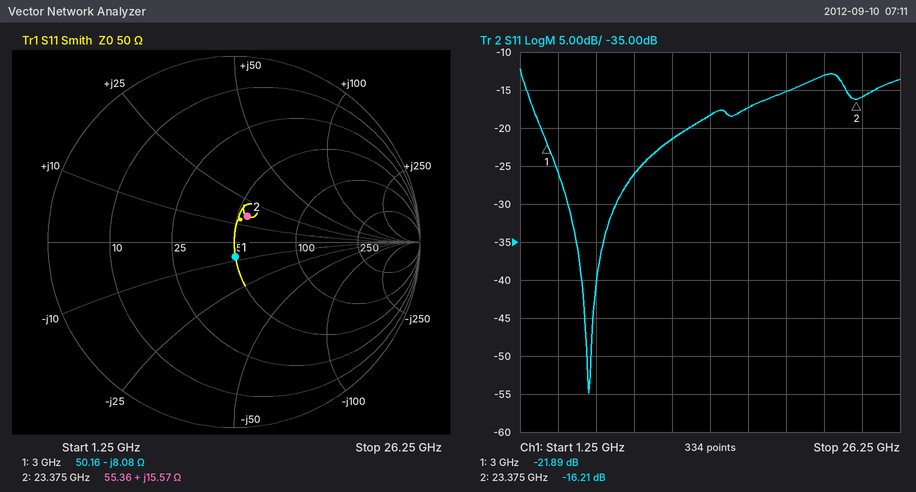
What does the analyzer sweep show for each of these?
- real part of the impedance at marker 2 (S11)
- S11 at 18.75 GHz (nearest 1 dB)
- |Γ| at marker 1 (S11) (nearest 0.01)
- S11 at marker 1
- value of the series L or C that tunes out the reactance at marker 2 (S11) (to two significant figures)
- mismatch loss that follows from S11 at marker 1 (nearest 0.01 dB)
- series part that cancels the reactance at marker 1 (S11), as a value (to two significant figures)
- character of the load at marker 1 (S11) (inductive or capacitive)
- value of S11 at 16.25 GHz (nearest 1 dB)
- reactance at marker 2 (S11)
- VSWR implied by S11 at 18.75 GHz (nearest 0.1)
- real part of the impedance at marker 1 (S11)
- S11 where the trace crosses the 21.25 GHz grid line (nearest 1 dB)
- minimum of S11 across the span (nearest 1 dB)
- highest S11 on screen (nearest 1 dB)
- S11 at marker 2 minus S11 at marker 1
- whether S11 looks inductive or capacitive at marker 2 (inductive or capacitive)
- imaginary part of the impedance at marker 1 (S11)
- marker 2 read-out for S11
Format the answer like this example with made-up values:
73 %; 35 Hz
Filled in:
55.36 Ω; -15 dB; 0.08; -21.89 dB; 440 fF; 0.03 dB; 430 pH; capacitive; -17 dB; +15.57 Ω; 1.4; 50.16 Ω; -13 dB; -55 dB; -12 dB; 5.68 dB; inductive; -8.08 Ω; -16.21 dB
